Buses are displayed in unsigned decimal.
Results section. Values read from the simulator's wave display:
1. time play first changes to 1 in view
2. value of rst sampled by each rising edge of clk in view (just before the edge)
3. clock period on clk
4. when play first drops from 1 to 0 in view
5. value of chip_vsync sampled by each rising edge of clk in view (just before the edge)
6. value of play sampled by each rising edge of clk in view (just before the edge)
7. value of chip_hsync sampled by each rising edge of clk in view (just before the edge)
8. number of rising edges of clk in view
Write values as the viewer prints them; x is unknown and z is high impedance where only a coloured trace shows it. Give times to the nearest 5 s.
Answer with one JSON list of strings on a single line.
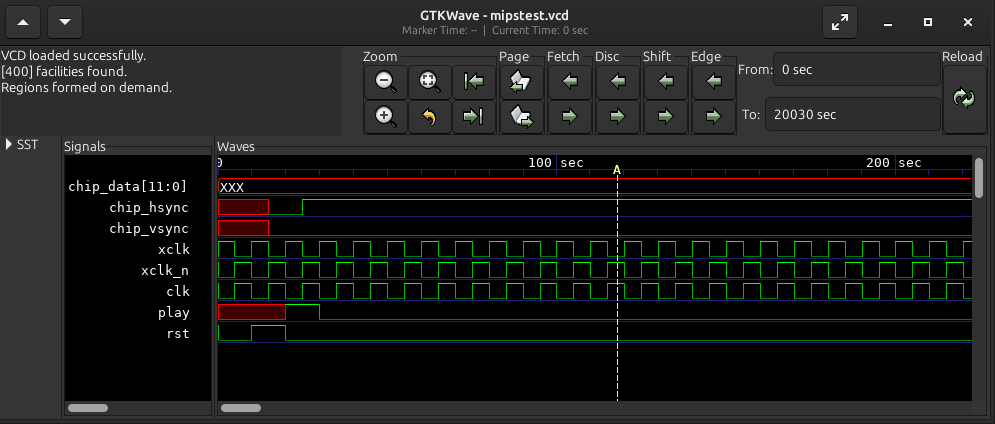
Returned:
["20 s", "0 1 0 0 0 0 0 0 0 0 0 0 0 0 0 0 0 0 0 0 0 0", "10 s", "30 s", "x x 0 0 0 0 0 0 0 0 0 0 0 0 0 0 0 0 0 0 0 0", "x x 1 0 0 0 0 0 0 0 0 0 0 0 0 0 0 0 0 0 0 0", "x x 0 1 1 1 1 1 1 1 1 1 1 1 1 1 1 1 1 1 1 1", "22"]
